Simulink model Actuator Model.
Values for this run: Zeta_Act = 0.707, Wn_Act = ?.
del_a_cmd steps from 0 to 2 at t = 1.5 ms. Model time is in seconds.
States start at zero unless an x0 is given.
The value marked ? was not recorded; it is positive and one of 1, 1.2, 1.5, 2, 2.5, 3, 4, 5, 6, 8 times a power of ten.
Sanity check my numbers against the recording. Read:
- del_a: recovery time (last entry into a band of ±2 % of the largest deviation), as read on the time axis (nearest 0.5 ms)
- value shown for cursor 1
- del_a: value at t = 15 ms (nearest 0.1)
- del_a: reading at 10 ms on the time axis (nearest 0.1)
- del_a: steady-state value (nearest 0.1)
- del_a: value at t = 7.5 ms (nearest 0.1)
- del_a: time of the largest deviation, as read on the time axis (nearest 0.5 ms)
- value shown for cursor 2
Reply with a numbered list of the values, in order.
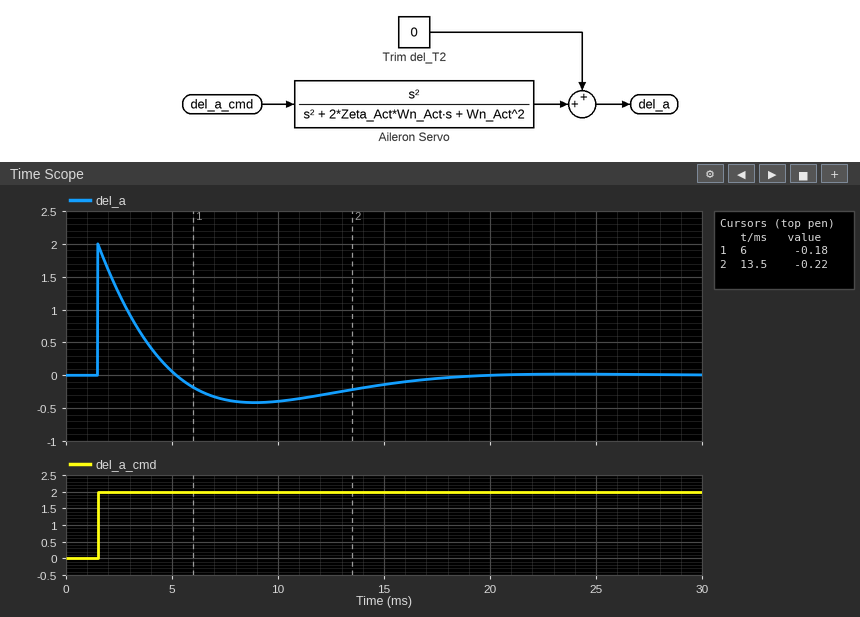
1. 18.0 ms
2. -0.18
3. -0.1
4. -0.4
5. 0.0
6. -0.4
7. 1.5 ms
8. -0.22
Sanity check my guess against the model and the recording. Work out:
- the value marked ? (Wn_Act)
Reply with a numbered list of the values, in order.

1. 300
